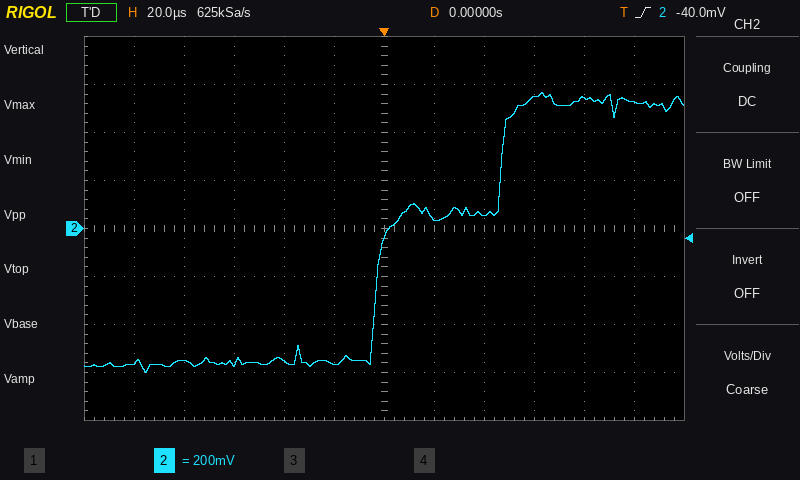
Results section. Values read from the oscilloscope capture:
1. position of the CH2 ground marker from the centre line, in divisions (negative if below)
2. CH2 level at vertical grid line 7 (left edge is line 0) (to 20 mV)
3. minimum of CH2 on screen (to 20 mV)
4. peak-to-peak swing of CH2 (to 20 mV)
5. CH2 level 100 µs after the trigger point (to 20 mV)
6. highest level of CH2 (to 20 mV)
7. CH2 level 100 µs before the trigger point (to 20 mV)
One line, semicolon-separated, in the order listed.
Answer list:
0.0 div; 40 mV; -600 mV; 1.16 V; 520 mV; 560 mV; -560 mV
